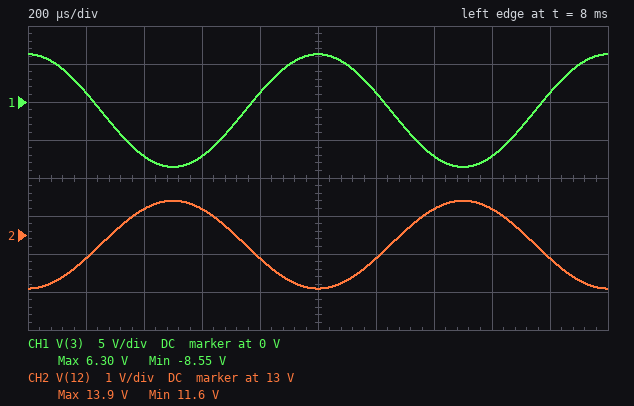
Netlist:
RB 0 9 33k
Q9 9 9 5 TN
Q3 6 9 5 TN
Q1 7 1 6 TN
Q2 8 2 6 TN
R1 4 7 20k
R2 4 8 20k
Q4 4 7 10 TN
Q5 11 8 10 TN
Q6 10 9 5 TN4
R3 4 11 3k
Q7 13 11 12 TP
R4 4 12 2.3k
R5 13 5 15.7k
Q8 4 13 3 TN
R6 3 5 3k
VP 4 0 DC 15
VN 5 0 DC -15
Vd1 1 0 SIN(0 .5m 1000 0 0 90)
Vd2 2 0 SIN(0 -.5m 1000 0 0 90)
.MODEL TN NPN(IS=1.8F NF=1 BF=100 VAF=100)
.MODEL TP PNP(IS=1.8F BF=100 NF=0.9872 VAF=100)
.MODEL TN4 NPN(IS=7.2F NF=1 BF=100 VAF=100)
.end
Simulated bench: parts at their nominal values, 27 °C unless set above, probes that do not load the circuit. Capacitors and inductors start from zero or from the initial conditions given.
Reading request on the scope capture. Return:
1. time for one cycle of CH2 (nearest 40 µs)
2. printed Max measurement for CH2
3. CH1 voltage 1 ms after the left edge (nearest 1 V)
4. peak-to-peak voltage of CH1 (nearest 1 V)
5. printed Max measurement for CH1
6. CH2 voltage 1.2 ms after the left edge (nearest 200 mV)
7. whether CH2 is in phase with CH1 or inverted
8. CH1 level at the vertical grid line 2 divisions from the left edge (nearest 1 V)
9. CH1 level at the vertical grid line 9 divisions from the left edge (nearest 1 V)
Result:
1.00 ms
13.9 V
6 V
15 V
6.30 V
12.4 V
inverted
-7 V
1 V
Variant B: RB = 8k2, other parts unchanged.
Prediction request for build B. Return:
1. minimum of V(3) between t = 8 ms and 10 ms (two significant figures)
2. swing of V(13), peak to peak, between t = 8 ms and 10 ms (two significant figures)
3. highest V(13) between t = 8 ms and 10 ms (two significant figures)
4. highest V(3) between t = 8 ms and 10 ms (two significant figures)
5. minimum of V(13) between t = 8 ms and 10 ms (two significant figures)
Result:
7.7 V
330 mV
8.8 V
8.0 V
8.4 V
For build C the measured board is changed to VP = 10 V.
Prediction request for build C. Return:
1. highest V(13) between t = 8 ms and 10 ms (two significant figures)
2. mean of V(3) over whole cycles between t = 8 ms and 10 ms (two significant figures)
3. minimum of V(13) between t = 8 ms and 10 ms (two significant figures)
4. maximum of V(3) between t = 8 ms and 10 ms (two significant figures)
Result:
6.2 V
-1.9 V
-8.5 V
5.4 V
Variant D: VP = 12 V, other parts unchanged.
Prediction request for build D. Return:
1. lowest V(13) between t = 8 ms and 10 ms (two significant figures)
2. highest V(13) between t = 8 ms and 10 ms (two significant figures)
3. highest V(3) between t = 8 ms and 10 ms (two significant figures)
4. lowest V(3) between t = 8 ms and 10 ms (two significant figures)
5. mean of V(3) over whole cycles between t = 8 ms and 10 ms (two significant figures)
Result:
-8.3 V
6.5 V
5.8 V
-9.0 V
-1.6 V
